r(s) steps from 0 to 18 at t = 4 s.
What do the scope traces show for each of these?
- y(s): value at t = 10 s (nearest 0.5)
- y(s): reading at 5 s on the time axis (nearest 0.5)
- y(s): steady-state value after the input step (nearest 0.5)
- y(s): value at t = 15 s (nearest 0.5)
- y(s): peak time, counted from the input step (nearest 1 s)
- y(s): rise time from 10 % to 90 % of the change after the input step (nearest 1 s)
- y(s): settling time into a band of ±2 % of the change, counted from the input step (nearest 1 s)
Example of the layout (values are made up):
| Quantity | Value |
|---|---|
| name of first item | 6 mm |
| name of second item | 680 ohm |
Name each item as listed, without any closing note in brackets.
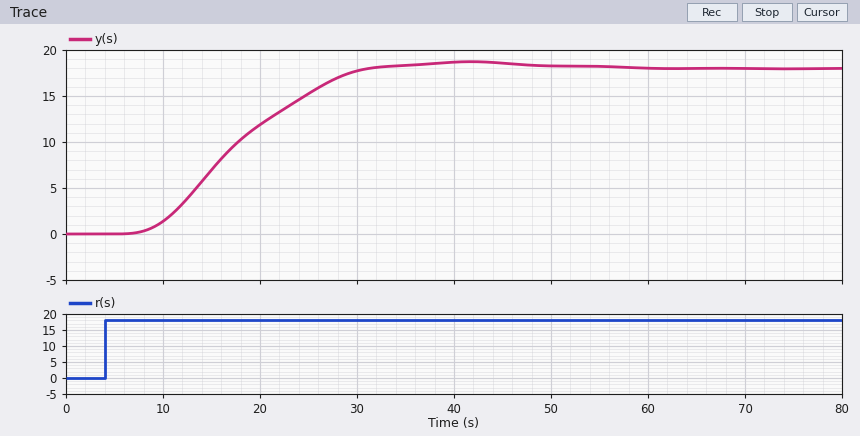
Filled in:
| Quantity | Value |
|---|---|
| y(s): value at t = 10 s | 1.5 |
| y(s): reading at 5 s on the time axis | 0.0 |
| y(s): steady-state value after the input step | 18.0 |
| y(s): value at t = 15 s | 7.0 |
| y(s): peak time, counted from the input step | 38 s |
| y(s): rise time from 10 % to 90 % of the change after the input step | 16 s |
| y(s): settling time into a band of ±2 % of the change, counted from the input step | 44 s |
